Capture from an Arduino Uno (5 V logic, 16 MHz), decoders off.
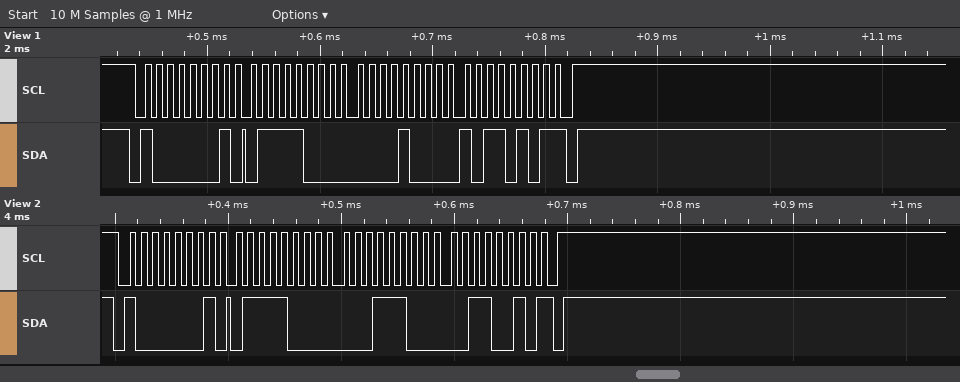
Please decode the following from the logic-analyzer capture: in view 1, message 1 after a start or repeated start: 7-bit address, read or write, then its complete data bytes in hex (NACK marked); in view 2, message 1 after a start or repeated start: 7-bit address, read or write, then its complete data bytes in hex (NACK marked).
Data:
0x40 read: 78 08 B5 NACK
0x40 read: 78 1C 32 NACK
